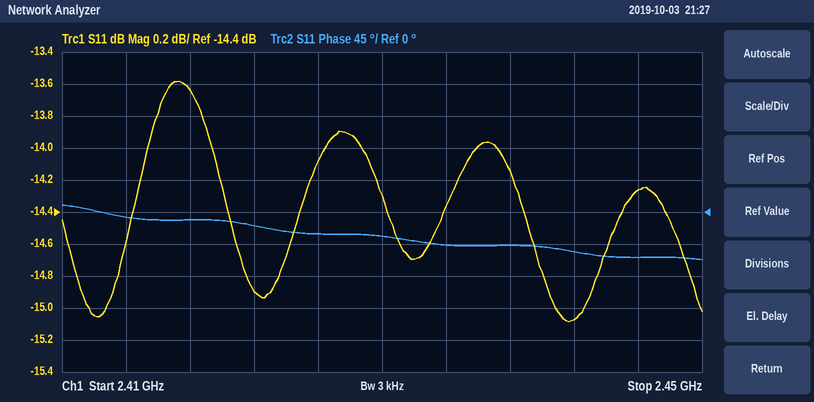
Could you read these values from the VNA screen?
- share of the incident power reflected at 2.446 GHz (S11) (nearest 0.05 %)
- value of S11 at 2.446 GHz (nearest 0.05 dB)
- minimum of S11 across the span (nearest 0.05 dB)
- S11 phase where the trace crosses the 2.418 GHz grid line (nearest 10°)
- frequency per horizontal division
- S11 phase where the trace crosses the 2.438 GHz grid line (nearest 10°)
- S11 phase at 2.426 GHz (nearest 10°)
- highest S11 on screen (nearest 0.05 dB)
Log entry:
3.75 %
-14.25 dB
-15.10 dB
-10°
4 MHz
-50°
-30°
-13.60 dB
